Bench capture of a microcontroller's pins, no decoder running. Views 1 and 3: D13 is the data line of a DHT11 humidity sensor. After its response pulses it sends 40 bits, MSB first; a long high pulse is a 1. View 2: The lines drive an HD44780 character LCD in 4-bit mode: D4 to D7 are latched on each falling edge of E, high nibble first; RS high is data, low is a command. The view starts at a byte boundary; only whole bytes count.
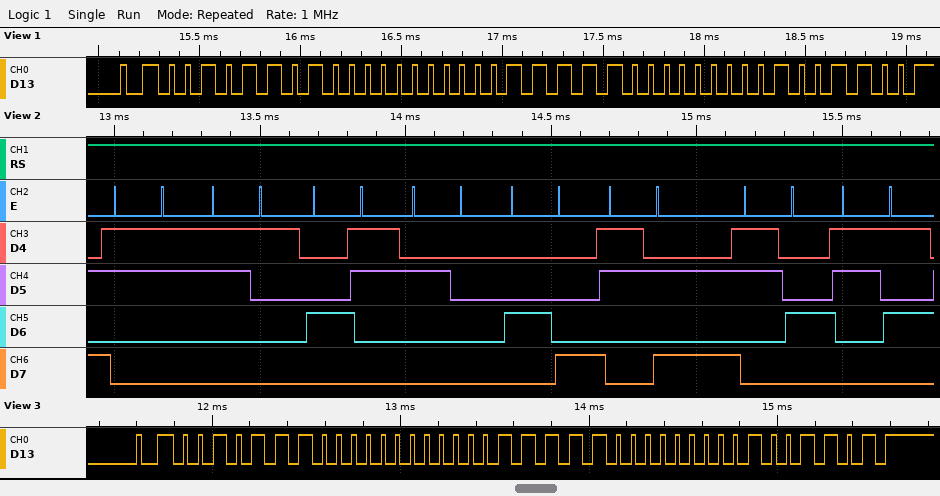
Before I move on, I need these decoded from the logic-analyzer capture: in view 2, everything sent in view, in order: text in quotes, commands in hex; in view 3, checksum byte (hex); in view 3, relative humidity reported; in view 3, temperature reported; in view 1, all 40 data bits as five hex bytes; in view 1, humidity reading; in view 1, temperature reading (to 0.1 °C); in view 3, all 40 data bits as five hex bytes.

"31C H:45"
0x4D
46 %
31.0 °C
2D 00 1F 00 4C
45 %
31.0 °C
2E 00 1F 00 4D
